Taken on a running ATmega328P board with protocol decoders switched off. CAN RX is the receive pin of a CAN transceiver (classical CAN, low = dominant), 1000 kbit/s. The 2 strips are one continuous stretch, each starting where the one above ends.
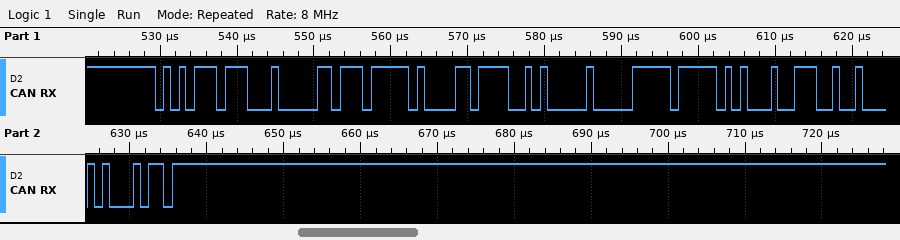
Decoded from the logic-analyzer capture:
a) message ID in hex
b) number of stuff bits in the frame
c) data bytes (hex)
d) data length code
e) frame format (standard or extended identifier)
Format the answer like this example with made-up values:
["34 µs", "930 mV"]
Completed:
["0x577", "6", "2E FC 37 94 00 FF D1 39", "8", "standard"]
